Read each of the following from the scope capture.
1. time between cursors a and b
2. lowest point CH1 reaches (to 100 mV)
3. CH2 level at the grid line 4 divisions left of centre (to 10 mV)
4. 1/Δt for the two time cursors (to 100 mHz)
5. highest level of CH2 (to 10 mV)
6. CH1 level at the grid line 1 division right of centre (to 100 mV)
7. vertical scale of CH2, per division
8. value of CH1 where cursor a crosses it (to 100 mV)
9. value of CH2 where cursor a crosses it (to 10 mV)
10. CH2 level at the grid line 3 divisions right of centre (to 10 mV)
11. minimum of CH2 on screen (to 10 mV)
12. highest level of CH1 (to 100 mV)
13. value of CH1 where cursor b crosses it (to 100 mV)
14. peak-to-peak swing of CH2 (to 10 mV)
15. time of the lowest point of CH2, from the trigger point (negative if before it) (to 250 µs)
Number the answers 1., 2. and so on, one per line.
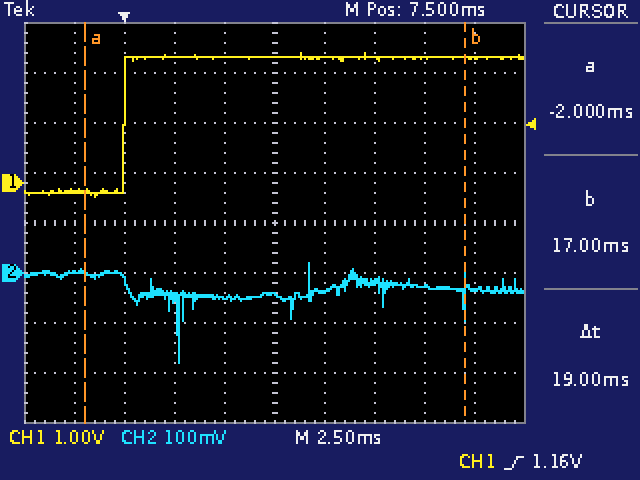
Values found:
1. 19 ms
2. -300 mV
3. 0 mV
4. 52.6 Hz
5. 20 mV
6. 2.5 V
7. 100 mV
8. -200 mV
9. 0 mV
10. -30 mV
11. -180 mV
12. 2.6 V
13. 2.5 V
14. 200 mV
15. +2.75 ms
